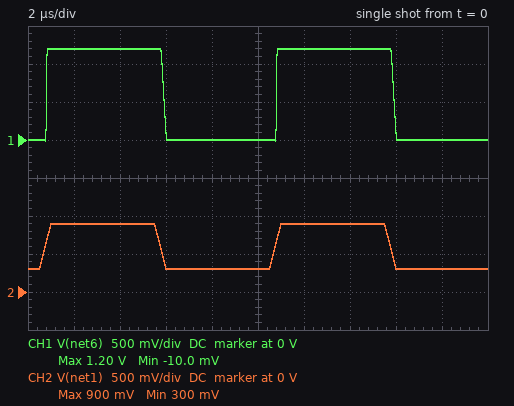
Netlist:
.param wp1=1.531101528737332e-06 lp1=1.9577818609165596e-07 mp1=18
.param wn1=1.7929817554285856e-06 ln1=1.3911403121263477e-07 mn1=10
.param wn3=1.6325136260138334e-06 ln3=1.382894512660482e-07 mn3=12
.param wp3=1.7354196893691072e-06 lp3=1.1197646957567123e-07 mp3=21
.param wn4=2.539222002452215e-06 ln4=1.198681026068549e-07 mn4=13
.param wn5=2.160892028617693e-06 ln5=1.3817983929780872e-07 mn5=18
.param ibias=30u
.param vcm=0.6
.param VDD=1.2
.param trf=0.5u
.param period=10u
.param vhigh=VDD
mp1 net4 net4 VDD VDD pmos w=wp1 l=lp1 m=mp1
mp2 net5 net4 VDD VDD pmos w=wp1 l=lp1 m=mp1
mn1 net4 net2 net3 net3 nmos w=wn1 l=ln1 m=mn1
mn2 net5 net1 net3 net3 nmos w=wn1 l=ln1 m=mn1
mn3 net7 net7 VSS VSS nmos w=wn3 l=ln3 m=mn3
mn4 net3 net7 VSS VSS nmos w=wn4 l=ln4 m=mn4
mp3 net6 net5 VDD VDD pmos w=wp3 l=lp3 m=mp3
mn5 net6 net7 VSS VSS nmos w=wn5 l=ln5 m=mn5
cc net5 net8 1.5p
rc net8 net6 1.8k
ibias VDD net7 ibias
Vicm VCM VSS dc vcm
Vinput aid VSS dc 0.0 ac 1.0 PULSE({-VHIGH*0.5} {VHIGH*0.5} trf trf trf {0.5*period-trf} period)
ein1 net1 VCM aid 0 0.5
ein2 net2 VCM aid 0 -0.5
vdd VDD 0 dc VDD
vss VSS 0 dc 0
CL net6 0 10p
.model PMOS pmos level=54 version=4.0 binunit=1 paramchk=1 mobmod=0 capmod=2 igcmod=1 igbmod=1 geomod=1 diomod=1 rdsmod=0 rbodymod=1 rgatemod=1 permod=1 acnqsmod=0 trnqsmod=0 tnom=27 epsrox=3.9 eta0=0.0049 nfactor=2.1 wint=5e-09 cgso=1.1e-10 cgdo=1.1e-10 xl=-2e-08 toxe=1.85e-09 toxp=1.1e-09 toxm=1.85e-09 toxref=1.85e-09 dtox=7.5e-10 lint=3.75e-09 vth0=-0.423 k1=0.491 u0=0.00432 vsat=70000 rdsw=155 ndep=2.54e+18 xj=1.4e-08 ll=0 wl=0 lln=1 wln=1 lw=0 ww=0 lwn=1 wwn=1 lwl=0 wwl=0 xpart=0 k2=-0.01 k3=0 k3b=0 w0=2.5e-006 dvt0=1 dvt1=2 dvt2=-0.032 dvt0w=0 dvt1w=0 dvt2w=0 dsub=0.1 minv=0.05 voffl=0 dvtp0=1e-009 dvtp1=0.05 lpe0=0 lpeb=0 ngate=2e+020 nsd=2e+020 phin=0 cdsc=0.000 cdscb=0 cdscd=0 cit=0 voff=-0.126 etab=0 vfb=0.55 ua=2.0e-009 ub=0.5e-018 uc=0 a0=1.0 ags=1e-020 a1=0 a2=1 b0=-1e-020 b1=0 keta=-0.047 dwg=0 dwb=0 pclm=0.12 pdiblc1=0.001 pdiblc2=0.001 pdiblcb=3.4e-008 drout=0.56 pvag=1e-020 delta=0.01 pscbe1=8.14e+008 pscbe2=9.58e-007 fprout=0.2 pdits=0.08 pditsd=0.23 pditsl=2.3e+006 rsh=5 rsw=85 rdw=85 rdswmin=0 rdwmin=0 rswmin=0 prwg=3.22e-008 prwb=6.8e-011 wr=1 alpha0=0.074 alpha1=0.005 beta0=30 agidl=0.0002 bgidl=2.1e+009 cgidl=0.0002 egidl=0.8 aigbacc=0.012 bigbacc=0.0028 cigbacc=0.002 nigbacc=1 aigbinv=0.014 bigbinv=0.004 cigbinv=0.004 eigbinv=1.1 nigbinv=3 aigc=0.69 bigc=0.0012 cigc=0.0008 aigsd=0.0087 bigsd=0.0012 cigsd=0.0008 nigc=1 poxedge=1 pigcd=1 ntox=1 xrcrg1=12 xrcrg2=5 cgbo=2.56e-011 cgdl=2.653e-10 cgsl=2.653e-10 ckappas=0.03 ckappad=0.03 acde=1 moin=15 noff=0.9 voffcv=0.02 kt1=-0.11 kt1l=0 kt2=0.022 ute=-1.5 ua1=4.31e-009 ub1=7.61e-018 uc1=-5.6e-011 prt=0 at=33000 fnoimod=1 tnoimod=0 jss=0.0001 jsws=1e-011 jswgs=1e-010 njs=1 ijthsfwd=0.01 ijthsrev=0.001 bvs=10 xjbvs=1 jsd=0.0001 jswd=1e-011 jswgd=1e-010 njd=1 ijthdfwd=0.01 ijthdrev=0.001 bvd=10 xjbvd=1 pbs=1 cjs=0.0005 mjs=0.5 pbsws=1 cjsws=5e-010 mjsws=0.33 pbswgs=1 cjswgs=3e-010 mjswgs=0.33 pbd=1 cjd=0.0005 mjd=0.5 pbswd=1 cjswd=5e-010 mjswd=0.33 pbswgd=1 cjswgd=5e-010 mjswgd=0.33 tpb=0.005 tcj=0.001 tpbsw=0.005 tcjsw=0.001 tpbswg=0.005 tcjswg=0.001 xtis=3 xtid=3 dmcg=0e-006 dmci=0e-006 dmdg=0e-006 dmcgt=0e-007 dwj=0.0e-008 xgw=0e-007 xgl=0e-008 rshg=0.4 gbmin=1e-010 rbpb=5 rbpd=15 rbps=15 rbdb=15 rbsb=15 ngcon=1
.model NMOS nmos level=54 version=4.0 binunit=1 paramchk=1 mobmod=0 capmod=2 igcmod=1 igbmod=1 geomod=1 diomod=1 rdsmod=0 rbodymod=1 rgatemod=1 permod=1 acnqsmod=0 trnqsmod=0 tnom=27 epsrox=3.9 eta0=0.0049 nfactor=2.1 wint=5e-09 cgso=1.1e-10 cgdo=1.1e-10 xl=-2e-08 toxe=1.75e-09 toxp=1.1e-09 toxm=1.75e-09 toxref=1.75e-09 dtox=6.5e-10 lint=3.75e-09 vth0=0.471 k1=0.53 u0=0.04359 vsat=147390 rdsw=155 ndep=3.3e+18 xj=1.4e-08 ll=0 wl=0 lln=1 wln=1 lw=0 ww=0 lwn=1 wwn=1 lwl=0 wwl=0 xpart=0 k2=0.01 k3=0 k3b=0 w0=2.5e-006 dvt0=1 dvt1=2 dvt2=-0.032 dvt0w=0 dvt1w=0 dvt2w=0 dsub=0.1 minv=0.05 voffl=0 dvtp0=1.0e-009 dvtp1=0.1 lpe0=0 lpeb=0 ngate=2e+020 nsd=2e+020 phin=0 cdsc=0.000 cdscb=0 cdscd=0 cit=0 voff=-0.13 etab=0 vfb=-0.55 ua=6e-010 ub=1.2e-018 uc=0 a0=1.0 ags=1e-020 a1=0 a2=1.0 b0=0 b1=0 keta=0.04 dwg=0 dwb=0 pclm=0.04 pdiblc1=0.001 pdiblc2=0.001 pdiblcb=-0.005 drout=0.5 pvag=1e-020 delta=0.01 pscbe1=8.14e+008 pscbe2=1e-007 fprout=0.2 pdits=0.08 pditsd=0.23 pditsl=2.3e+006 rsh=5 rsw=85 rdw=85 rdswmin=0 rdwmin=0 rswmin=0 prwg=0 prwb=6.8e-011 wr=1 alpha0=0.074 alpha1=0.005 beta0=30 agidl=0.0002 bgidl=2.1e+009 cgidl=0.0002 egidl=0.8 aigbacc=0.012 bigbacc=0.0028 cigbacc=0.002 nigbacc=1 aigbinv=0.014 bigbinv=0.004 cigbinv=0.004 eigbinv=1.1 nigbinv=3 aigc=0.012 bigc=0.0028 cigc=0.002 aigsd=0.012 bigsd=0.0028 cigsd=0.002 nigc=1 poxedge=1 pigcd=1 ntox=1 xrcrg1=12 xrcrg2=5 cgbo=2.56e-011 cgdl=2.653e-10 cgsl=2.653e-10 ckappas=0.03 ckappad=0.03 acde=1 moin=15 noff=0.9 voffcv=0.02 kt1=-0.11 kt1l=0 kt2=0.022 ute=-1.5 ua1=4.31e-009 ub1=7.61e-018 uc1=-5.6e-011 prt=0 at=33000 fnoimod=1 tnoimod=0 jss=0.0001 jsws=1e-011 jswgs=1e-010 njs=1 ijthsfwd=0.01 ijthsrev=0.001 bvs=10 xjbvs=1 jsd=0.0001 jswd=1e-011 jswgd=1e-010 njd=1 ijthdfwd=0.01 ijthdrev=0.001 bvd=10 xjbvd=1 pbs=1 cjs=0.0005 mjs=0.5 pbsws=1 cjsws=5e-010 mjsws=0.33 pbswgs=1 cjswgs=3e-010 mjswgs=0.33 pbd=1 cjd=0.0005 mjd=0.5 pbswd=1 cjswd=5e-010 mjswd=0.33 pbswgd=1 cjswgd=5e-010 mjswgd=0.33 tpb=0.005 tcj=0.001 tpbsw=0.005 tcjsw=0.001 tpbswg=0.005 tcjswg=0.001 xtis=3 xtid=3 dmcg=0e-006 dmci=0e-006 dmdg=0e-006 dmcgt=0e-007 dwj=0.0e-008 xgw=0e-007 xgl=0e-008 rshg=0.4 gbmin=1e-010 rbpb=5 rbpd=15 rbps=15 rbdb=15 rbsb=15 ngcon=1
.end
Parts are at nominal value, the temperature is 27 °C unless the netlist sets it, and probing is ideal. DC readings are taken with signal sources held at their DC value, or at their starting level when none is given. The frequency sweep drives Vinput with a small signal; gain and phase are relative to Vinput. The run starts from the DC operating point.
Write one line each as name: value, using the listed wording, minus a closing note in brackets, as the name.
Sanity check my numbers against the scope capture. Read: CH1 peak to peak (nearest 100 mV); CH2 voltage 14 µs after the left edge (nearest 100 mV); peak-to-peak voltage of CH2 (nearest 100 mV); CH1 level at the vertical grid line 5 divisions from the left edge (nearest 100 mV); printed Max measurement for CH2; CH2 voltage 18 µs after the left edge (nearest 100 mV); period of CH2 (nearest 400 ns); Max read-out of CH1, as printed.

CH1 peak to peak: 1.2 V
CH2 voltage 14 µs after the left edge: 900 mV
peak-to-peak voltage of CH2: 600 mV
CH1 level at the vertical grid line 5 divisions from the left edge: 0 V
printed Max measurement for CH2: 900 mV
CH2 voltage 18 µs after the left edge: 300 mV
period of CH2: 10.0 µs
Max read-out of CH1, as printed: 1.20 V
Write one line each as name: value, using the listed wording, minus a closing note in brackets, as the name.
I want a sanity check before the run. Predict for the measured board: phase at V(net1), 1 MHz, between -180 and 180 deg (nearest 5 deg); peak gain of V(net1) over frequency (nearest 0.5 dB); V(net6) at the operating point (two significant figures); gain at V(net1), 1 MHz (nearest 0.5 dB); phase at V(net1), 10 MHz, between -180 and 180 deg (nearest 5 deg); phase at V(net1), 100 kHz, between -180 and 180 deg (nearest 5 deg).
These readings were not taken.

phase at V(net1), 1 MHz, between -180 and 180 deg: 0 deg
peak gain of V(net1) over frequency: -6.0 dB
V(net6) at the operating point: 1.1 V
gain at V(net1), 1 MHz: -6.0 dB
phase at V(net1), 10 MHz, between -180 and 180 deg: 0 deg
phase at V(net1), 100 kHz, between -180 and 180 deg: 0 deg
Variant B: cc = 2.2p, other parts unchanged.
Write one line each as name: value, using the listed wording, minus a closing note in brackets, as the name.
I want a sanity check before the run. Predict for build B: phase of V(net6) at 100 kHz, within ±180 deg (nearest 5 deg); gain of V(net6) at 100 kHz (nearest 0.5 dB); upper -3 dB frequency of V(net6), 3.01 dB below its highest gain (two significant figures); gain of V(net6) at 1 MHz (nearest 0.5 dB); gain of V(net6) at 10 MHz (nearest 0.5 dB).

phase of V(net6) at 100 kHz, within ±180 deg: -40 deg
gain of V(net6) at 100 kHz: 45.5 dB
upper -3 dB frequency of V(net6), 3.01 dB below its highest gain: 130 kHz
gain of V(net6) at 1 MHz: 29.5 dB
gain of V(net6) at 10 MHz: 8.5 dB
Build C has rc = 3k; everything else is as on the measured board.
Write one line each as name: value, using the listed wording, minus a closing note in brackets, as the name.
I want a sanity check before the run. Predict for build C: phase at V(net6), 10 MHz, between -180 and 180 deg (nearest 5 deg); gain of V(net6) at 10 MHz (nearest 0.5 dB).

phase at V(net6), 10 MHz, between -180 and 180 deg: -110 deg
gain of V(net6) at 10 MHz: 12.0 dB
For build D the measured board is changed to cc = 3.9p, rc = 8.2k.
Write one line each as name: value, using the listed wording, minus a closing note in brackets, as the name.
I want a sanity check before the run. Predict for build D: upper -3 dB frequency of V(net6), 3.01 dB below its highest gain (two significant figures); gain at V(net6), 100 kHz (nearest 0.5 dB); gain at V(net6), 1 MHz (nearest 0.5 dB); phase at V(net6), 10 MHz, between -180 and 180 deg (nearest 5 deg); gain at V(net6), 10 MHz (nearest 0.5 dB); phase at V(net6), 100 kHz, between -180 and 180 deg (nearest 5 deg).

upper -3 dB frequency of V(net6), 3.01 dB below its highest gain: 72 kHz
gain at V(net6), 100 kHz: 43.0 dB
gain at V(net6), 1 MHz: 24.5 dB
phase at V(net6), 10 MHz, between -180 and 180 deg: -60 deg
gain at V(net6), 10 MHz: 9.5 dB
phase at V(net6), 100 kHz, between -180 and 180 deg: -55 deg
